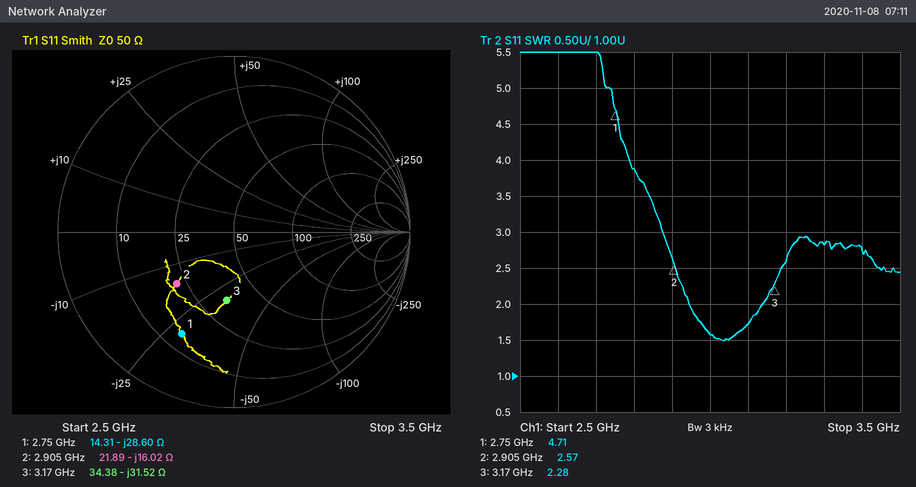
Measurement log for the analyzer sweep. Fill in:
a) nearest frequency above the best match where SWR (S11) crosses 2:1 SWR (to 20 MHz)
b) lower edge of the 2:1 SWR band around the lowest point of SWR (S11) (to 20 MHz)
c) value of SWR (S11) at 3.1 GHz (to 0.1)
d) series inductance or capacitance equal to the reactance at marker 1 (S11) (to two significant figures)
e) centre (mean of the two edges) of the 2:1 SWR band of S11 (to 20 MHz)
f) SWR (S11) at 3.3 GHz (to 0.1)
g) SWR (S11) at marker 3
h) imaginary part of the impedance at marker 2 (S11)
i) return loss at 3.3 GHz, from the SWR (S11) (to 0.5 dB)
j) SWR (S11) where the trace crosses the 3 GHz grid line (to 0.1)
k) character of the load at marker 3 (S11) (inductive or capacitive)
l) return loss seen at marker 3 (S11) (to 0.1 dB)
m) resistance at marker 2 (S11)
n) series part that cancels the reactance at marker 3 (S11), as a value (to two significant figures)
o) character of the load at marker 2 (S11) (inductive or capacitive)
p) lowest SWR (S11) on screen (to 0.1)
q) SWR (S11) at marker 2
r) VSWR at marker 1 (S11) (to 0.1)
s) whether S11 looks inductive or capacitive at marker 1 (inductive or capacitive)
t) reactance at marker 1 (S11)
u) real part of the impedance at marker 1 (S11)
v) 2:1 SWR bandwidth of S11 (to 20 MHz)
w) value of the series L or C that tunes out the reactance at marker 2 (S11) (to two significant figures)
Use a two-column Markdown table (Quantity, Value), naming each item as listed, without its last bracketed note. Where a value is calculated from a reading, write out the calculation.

| Quantity | Value |
|---|---|
| nearest frequency above the best match where SWR (S11) crosses 2:1 SWR | 3.14 GHz |
| lower edge of the 2:1 SWR band around the lowest point of SWR (S11) | 2.94 GHz |
| value of SWR (S11) at 3.1 GHz | 1.7 |
| series inductance or capacitance equal to the reactance at marker 1 (S11) | C = 1/(2π × 2.75 GHz × 28.6 Ω) ≈ 2.0 pF |
| centre (mean of the two edges) of the 2:1 SWR band of S11 | 3.04 GHz |
| SWR (S11) at 3.3 GHz | 2.8 |
| SWR (S11) at marker 3 | 2.28 |
| imaginary part of the impedance at marker 2 | -16.02 Ω |
| return loss at 3.3 GHz, from the SWR (S11) | −20 log10((2.8 − 1)/(2.8 + 1)) ≈ 6.5 dB |
| SWR (S11) where the trace crosses the 3 GHz grid line | 1.6 |
| character of the load at marker 3 (S11) | capacitive |
| return loss seen at marker 3 (S11) | 8.2 dB |
| resistance at marker 2 | 21.89 Ω |
| series part that cancels the reactance at marker 3 (S11), as a value | L = 31.52 Ω/(2π × 3.17 GHz) ≈ 1.6 nH |
| character of the load at marker 2 (S11) | capacitive |
| lowest SWR (S11) on screen | 1.5 |
| SWR (S11) at marker 2 | 2.57 |
| VSWR at marker 1 (S11) | 4.7 |
| whether S11 looks inductive or capacitive at marker 1 | capacitive |
| reactance at marker 1 | -28.60 Ω |
| real part of the impedance at marker 1 | 14.31 Ω |
| 2:1 SWR bandwidth of S11 | 3.14 GHz − 2.94 GHz = 200 MHz |
| value of the series L or C that tunes out the reactance at marker 2 (S11) | L = 16.02 Ω/(2π × 2.905 GHz) ≈ 878 pH, so 880 pH to two significant figures |
